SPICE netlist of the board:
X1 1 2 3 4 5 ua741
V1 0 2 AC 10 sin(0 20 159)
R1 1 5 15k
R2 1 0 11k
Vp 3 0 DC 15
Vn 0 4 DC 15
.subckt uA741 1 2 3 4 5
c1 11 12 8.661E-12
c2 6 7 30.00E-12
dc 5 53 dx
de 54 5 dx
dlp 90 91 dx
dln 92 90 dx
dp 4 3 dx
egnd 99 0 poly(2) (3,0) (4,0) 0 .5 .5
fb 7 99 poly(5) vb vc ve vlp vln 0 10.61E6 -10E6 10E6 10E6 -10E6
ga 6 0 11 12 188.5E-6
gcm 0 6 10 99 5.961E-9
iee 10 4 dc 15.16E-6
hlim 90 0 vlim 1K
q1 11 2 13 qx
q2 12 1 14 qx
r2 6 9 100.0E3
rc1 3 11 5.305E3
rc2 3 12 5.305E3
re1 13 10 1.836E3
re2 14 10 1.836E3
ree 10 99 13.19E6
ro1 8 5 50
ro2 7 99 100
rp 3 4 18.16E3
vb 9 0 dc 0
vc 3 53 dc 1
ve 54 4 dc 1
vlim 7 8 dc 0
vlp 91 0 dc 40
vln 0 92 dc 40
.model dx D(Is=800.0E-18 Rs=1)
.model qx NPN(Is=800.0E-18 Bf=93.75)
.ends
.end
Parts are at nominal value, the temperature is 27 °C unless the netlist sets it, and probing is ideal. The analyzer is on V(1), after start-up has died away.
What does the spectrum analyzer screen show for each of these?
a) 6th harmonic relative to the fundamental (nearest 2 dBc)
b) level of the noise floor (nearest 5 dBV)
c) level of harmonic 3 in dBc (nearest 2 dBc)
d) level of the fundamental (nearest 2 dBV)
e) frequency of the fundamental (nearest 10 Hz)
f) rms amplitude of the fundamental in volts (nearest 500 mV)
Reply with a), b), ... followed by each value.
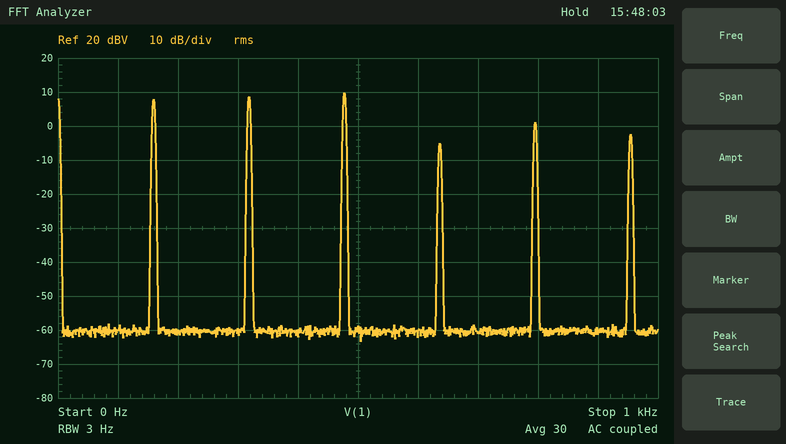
a) -10 dBc
b) -60 dBV
c) 2 dBc
d) 8 dBV
e) 160 Hz
f) 2.5 V
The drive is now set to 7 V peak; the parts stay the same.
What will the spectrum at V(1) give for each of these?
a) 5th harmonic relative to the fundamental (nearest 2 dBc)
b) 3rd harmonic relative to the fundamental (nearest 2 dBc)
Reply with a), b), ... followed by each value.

a) -14 dBc
b) -10 dBc
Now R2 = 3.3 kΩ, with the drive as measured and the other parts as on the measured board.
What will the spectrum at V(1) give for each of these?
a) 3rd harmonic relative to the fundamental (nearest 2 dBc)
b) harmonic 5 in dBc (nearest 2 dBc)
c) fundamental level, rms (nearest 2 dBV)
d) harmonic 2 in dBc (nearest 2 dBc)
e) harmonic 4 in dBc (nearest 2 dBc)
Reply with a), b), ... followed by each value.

a) 4 dBc
b) -4 dBc
c) 0 dBV
d) 2 dBc
e) -12 dBc
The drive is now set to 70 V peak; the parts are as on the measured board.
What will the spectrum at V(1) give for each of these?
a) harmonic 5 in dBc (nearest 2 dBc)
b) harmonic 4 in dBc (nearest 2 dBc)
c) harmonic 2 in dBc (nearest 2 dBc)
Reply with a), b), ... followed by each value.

a) 2 dBc
b) 6 dBc
c) 6 dBc
